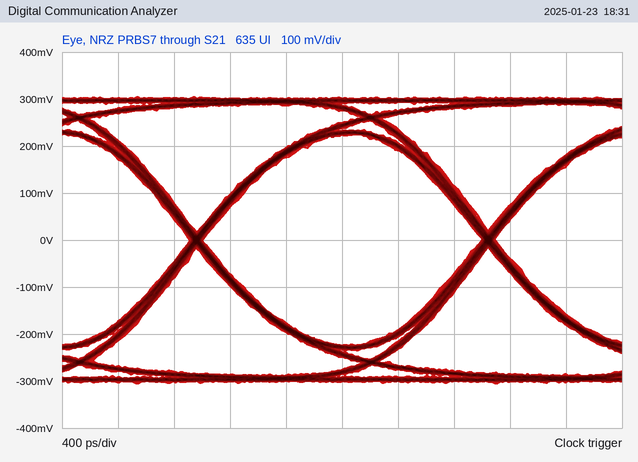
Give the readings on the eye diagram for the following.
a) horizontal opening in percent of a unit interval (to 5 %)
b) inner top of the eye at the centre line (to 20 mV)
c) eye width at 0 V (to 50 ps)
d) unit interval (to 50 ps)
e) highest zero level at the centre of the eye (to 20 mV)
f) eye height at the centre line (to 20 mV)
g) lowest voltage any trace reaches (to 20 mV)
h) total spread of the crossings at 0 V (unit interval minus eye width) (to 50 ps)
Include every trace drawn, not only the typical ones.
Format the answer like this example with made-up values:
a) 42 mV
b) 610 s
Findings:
a) 95 %
b) 220 mV
c) 2.00 ns
d) 2.10 ns
e) -220 mV
f) 440 mV
g) -300 mV
h) 100 ps
